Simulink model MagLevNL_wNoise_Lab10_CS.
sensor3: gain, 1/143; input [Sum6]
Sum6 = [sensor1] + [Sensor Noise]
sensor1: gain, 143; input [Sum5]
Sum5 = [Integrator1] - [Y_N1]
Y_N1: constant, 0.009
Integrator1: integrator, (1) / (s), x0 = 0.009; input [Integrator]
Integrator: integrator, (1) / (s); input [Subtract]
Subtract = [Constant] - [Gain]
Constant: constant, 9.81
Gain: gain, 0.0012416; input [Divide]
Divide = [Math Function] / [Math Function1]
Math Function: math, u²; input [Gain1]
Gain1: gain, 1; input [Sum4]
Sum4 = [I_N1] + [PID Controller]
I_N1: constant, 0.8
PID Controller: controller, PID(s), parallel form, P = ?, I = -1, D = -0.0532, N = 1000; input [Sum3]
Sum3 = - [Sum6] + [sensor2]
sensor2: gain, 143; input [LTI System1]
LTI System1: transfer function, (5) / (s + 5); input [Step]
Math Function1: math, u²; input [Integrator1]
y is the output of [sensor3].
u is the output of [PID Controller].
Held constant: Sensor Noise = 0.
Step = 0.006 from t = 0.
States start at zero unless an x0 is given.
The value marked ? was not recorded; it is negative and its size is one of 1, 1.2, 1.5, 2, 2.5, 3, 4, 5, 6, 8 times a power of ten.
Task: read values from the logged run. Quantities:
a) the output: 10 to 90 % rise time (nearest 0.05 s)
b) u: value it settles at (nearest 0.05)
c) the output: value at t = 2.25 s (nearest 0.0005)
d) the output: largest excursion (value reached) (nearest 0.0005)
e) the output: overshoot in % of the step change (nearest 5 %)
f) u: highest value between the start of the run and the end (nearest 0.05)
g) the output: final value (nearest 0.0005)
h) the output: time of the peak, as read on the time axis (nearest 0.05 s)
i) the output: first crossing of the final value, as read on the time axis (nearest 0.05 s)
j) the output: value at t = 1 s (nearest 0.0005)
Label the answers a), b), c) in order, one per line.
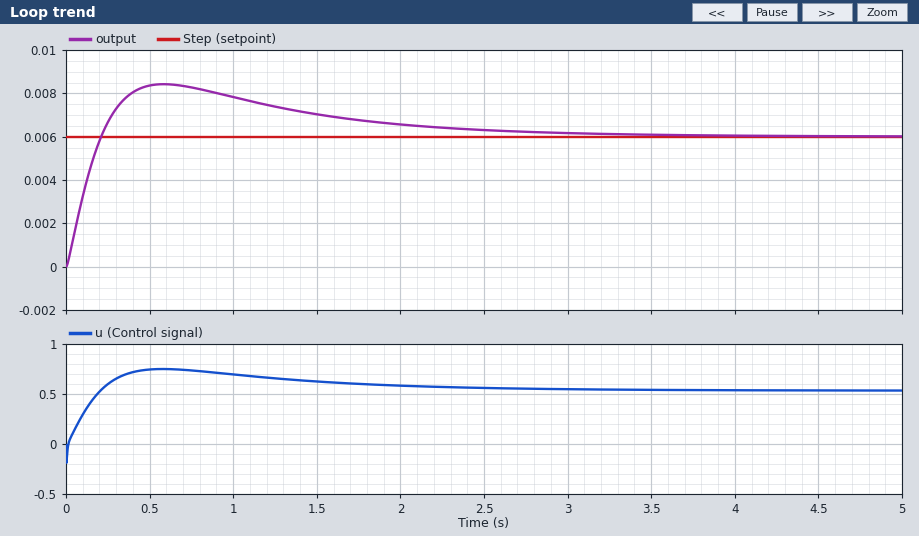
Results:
a) 0.15 s
b) 0.55
c) 0.0065
d) 0.0085
e) 40 %
f) 0.75
g) 0.0060
h) 0.60 s
i) 0.20 s
j) 0.0080
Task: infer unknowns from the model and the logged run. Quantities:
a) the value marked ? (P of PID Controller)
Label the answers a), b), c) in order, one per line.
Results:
a) -1.5
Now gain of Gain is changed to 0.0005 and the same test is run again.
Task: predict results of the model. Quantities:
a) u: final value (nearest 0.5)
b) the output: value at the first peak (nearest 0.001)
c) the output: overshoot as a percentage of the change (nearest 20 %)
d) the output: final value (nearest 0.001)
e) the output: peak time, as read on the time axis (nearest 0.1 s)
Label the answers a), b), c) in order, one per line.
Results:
a) 1.5
b) 0.016
c) 160 %
d) 0.006
e) 0.4 s
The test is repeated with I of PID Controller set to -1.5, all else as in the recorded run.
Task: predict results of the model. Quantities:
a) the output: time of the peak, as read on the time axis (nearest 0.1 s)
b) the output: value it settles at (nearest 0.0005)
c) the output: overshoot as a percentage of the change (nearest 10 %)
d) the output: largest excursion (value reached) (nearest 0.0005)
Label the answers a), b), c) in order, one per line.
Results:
a) 0.5 s
b) 0.0060
c) 30 %
d) 0.0080
